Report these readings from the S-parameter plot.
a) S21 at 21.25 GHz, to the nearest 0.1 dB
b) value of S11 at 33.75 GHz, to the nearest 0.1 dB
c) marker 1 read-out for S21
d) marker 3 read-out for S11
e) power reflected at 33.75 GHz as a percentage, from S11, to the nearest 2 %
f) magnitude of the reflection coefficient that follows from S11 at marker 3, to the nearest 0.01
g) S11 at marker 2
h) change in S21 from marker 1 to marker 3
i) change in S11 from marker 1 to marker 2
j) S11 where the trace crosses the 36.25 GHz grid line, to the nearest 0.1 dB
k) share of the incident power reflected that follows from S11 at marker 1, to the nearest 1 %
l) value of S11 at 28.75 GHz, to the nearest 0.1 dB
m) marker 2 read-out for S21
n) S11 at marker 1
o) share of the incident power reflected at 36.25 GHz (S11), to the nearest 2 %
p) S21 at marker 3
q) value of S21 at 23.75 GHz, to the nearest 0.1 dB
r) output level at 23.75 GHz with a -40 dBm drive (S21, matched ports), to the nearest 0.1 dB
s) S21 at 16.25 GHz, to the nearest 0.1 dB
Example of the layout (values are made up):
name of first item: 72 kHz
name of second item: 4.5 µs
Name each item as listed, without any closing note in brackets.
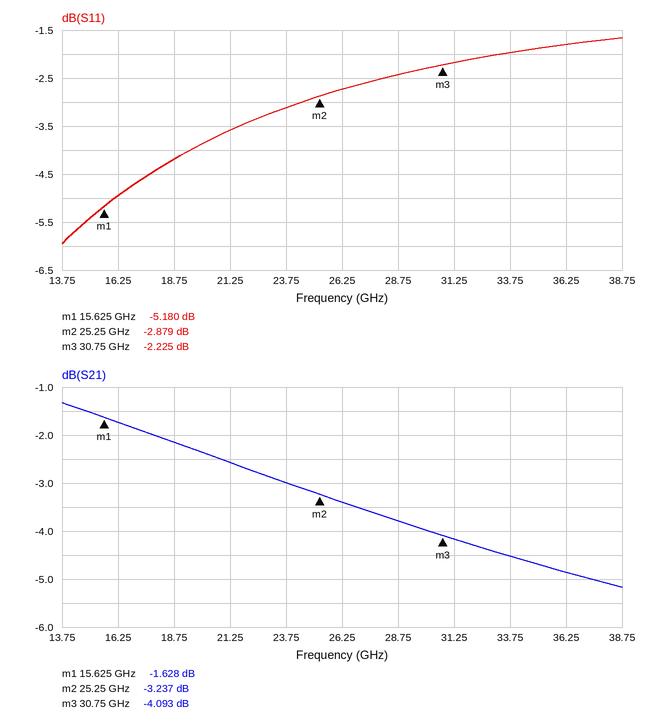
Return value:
S21 at 21.25 GHz, to the nearest 0.1 dB: -2.6 dB
value of S11 at 33.75 GHz, to the nearest 0.1 dB: -2.0 dB
marker 1 read-out for S21: -1.628 dB
marker 3 read-out for S11: -2.225 dB
power reflected at 33.75 GHz as a percentage, from S11, to the nearest 2 %: 64 %
magnitude of the reflection coefficient that follows from S11 at marker 3, to the nearest 0.01: 0.77
S11 at marker 2: -2.879 dB
change in S21 from marker 1 to marker 3: -2.465 dB
change in S11 from marker 1 to marker 2: 2.301 dB
S11 where the trace crosses the 36.25 GHz grid line, to the nearest 0.1 dB: -1.8 dB
share of the incident power reflected that follows from S11 at marker 1, to the nearest 1 %: 30 %
value of S11 at 28.75 GHz, to the nearest 0.1 dB: -2.4 dB
marker 2 read-out for S21: -3.237 dB
S11 at marker 1: -5.180 dB
share of the incident power reflected at 36.25 GHz (S11), to the nearest 2 %: 66 %
S21 at marker 3: -4.093 dB
value of S21 at 23.75 GHz, to the nearest 0.1 dB: -3.0 dB
output level at 23.75 GHz with a -40 dBm drive (S21, matched ports), to the nearest 0.1 dB: -43.0 dBm
S21 at 16.25 GHz, to the nearest 0.1 dB: -1.7 dB
